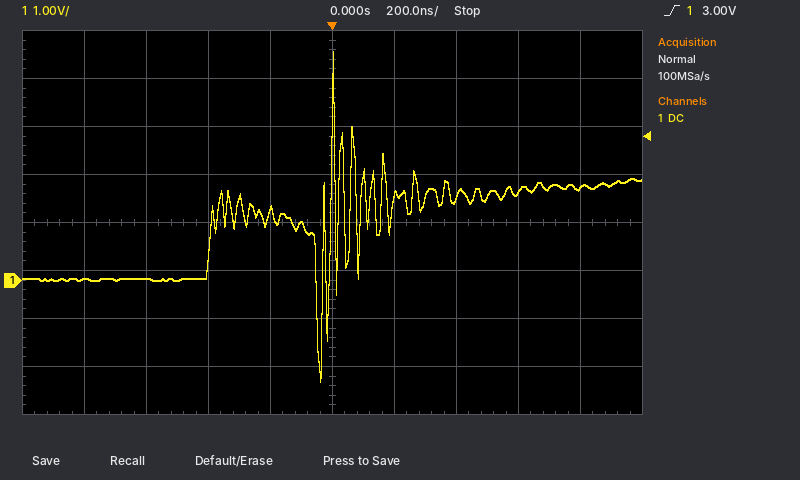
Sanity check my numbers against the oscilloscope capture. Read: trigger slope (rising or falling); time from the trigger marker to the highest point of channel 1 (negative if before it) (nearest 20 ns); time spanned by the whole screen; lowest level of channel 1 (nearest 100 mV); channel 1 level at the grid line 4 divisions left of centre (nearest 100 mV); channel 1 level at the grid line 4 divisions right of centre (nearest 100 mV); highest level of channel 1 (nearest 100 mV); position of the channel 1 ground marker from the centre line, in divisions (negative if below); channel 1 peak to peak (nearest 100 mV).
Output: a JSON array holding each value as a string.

["rising", "0 ns", "2 µs", "-2.1 V", "0.0 V", "1.9 V", "4.8 V", "-1.2 div", "6.9 V"]
